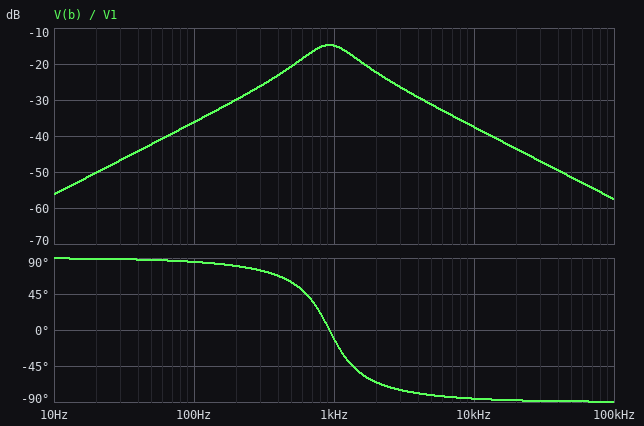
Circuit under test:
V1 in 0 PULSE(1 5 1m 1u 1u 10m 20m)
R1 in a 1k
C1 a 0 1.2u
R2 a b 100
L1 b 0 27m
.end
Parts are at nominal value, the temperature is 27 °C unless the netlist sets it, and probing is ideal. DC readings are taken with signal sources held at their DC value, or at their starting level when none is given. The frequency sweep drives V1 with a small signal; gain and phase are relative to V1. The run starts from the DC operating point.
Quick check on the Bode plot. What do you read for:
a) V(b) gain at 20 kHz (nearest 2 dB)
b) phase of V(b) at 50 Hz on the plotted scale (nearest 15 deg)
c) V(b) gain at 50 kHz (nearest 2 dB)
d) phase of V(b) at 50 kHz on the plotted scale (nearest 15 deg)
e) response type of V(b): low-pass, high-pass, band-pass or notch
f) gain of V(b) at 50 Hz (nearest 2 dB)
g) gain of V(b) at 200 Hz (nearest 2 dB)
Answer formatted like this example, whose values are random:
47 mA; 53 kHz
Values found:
-44 dB; 90 deg; -52 dB; -90 deg; band-pass; -42 dB; -30 dB
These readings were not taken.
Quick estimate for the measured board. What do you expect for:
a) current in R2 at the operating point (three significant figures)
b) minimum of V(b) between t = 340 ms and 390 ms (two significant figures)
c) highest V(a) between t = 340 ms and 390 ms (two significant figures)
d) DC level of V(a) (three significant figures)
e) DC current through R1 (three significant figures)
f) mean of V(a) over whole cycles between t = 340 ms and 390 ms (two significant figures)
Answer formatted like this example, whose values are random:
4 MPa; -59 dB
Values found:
909 µA; -350 mV; 710 mV; 90.9 mV; 909 µA; 270 mV
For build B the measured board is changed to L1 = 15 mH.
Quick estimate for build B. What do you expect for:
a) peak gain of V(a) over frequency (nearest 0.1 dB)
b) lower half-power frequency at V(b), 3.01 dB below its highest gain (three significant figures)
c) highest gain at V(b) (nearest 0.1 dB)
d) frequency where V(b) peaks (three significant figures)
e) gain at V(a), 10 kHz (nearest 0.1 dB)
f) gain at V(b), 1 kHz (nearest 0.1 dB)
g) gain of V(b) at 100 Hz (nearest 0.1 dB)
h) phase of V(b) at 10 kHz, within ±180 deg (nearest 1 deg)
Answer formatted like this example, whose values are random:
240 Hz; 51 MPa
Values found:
-16.5 dB; 783 Hz; -19.1 dB; 1.24 kHz; -37.4 dB; -19.9 dB; -41.3 dB; -83 deg
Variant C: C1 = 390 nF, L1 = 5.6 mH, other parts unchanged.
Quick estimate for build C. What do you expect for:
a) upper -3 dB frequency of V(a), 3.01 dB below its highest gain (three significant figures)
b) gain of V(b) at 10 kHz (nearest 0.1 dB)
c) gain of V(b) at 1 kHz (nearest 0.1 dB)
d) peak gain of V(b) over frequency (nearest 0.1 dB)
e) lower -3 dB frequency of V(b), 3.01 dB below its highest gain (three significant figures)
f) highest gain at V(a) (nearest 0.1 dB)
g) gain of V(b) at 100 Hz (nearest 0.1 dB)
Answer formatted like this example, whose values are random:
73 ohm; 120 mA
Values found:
5.00 kHz; -27.2 dB; -29.5 dB; -18.0 dB; 2.30 kHz; -15.7 dB; -49.9 dB
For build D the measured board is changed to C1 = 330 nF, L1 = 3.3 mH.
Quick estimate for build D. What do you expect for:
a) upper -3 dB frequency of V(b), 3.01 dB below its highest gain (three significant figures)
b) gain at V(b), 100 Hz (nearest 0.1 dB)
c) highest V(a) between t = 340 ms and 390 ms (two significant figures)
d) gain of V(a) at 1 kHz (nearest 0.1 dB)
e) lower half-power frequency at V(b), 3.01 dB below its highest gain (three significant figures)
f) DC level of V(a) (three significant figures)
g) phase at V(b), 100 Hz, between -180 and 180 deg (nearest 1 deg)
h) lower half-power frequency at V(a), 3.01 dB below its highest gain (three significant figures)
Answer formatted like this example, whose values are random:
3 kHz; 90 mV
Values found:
8.36 kHz; -54.5 dB; 560 mV; -20.5 dB; 3.06 kHz; 90.9 mV; 89 deg; 612 Hz
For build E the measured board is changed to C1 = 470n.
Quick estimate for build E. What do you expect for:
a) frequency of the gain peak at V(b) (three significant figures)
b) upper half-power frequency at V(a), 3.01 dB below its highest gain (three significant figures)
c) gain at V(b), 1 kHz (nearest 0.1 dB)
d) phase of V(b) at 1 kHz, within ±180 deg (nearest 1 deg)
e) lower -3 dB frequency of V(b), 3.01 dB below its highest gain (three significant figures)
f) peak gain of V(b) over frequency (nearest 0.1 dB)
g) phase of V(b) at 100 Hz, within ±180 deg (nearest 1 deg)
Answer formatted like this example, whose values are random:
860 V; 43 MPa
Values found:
1.48 kHz; 1.98 kHz; -13.0 dB; 52 deg; 1.09 kHz; -8.8 dB; 88 deg
